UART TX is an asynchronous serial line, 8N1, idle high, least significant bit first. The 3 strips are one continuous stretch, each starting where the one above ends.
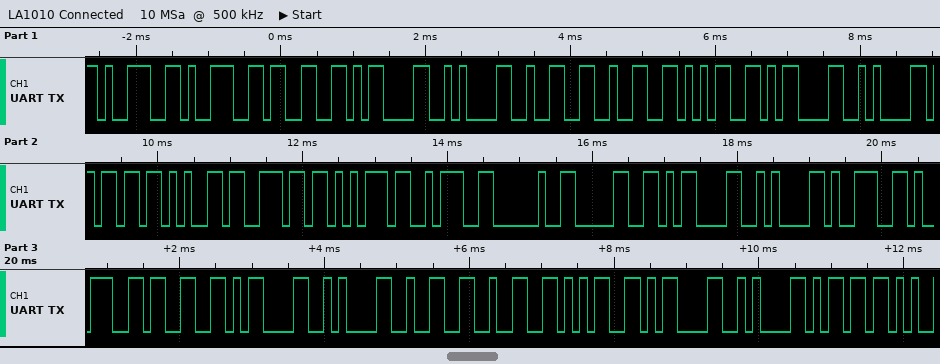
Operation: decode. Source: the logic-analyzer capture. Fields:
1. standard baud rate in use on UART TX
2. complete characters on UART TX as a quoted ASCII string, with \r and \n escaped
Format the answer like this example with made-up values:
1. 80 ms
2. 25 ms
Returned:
1. 9600 baud
2. "993\r\n225\r\nmenu: 0\r\n993\r\n225\r\nm"
